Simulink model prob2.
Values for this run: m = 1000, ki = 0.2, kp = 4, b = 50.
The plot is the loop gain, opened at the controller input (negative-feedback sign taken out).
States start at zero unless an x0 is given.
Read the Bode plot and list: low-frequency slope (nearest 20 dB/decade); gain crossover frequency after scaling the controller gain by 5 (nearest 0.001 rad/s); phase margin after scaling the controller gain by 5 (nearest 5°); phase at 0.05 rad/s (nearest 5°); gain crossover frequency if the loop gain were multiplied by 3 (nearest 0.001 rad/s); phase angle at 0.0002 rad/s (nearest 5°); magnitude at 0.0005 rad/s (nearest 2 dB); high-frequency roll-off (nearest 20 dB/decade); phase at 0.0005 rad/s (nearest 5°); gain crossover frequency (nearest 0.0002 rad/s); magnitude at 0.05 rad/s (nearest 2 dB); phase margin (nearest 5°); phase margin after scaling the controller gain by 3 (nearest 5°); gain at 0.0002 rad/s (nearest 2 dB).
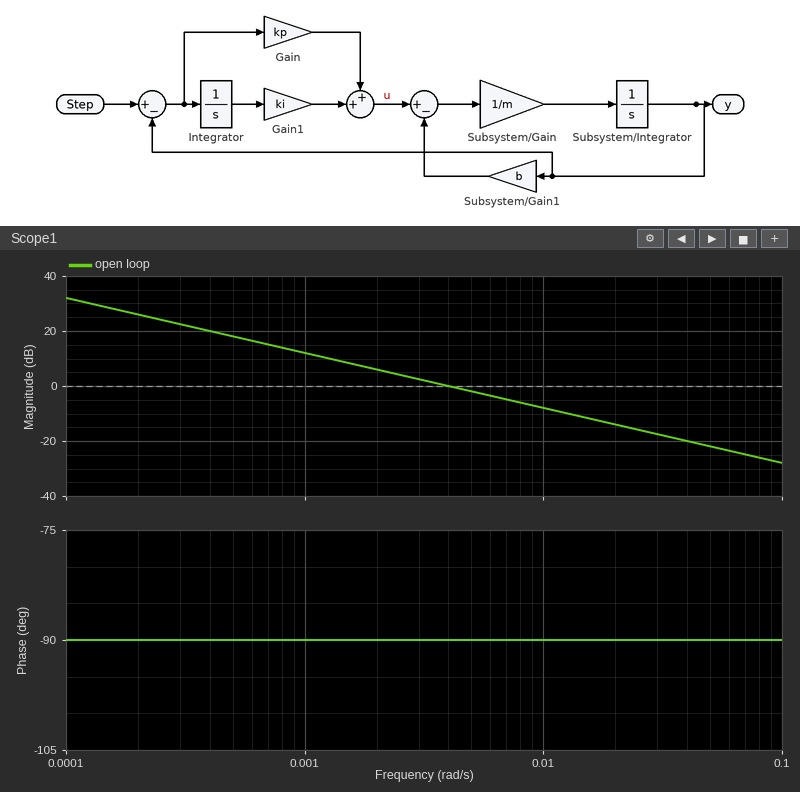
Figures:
-20 dB/decade
0.020 rad/s
90°
-90°
0.012 rad/s
-90°
18 dB
-20 dB/decade
-90°
0.0040 rad/s
-22 dB
90°
90°
26 dB
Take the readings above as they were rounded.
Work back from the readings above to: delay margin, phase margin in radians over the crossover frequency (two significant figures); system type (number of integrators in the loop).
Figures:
390 s
1
